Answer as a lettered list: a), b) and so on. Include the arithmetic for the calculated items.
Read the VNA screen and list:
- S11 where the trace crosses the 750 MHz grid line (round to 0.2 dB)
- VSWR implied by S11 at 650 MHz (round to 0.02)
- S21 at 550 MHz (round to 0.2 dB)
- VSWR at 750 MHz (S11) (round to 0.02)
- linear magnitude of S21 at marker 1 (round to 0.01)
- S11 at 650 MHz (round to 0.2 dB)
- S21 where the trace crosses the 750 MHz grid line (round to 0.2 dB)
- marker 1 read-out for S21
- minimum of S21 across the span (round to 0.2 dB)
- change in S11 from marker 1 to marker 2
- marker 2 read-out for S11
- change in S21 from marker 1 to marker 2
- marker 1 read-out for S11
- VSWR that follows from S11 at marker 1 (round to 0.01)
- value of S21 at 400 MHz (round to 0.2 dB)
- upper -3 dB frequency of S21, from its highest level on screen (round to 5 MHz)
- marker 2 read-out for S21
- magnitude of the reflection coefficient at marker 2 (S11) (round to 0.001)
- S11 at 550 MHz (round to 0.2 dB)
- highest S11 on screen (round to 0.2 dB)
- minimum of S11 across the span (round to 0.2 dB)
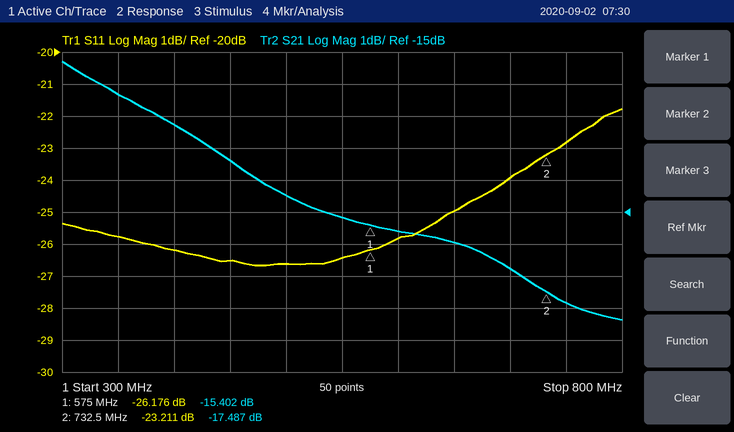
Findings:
a) -22.8 dB
b) |Γ| = 10^(-25/20) = 0.0562; VSWR = (1 + 0.0562)/(1 − 0.0562) ≈ 1.12
c) -15.2 dB
d) |Γ| = 10^(-22.8/20) = 0.0724; VSWR = (1 + 0.0724)/(1 − 0.0724) ≈ 1.16
e) 10^(-15.402/20) ≈ 0.17
f) -25.0 dB
g) -17.8 dB
h) -15.402 dB
i) -18.4 dB
j) -23.211 − (-26.176) = 2.965 dB
k) -23.211 dB
l) -17.487 − (-15.402) = -2.085 dB
m) -26.176 dB
n) (1 + 0.0491)/(1 − 0.0491) ≈ 1.10
o) -12.2 dB
p) 445 MHz
q) -17.487 dB
r) 10^(-23.211/20) ≈ 0.069
s) -26.4 dB
t) -21.8 dB
u) -26.6 dB
